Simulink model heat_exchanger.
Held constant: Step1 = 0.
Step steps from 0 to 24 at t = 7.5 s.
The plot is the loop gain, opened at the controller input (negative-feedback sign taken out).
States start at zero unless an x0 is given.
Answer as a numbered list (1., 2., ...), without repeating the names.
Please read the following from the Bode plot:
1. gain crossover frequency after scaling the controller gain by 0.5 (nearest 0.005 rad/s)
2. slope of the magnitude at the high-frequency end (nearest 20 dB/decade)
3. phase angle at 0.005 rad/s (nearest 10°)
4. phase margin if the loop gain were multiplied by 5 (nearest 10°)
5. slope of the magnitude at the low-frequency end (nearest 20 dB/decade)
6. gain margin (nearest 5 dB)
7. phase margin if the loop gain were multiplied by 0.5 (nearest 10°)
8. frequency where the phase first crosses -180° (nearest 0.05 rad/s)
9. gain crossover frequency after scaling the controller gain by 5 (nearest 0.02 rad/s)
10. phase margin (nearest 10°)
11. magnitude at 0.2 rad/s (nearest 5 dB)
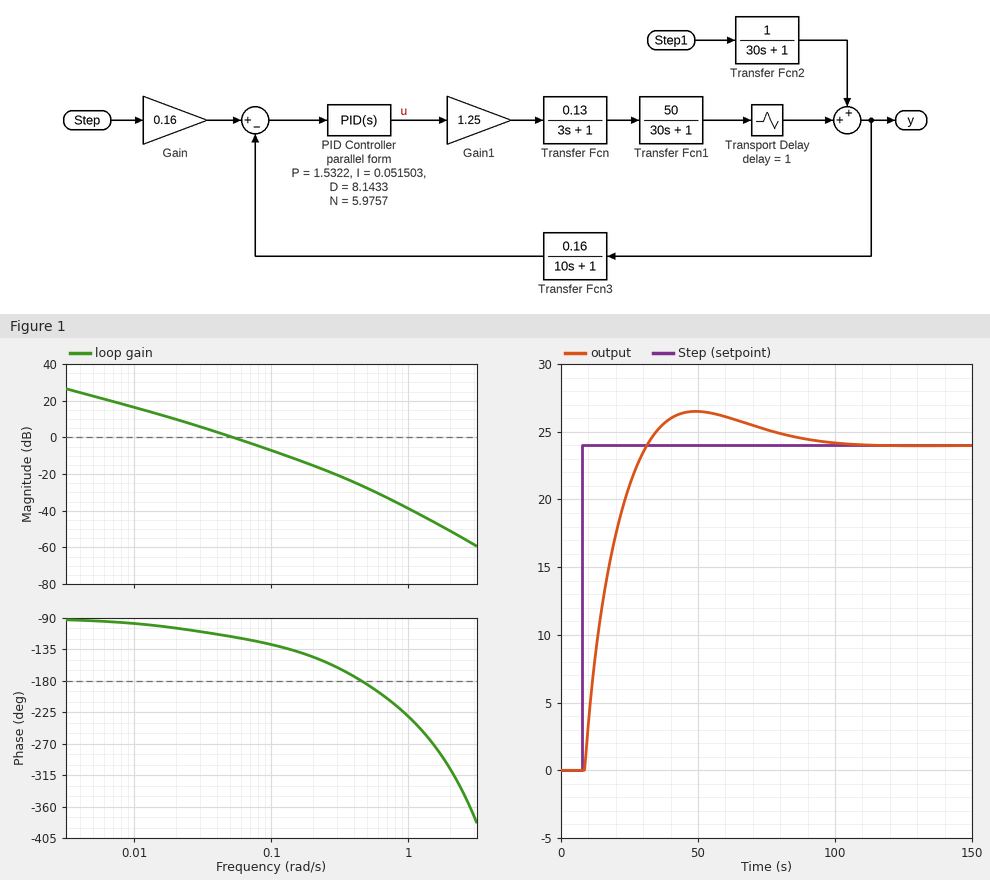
1. 0.030 rad/s
2. -40 dB/decade
3. -90°
4. 40°
5. -20 dB/decade
6. 25 dB
7. 70°
8. 0.45 rad/s
9. 0.18 rad/s
10. 60°
11. -15 dB
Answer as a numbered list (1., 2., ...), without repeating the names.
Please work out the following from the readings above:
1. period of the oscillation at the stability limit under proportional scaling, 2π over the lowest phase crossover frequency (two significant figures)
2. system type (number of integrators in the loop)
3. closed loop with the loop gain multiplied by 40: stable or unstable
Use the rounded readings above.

1. 14 s
2. 1
3. unstable
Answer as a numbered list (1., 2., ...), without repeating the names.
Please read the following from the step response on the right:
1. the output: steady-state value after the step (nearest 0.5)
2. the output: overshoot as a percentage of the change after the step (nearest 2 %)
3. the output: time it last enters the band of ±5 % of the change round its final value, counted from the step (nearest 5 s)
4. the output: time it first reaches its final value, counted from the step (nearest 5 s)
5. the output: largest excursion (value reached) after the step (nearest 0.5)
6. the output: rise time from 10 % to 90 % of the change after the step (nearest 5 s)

1. 24.0
2. 10 %
3. 65 s
4. 25 s
5. 26.5
6. 15 s
